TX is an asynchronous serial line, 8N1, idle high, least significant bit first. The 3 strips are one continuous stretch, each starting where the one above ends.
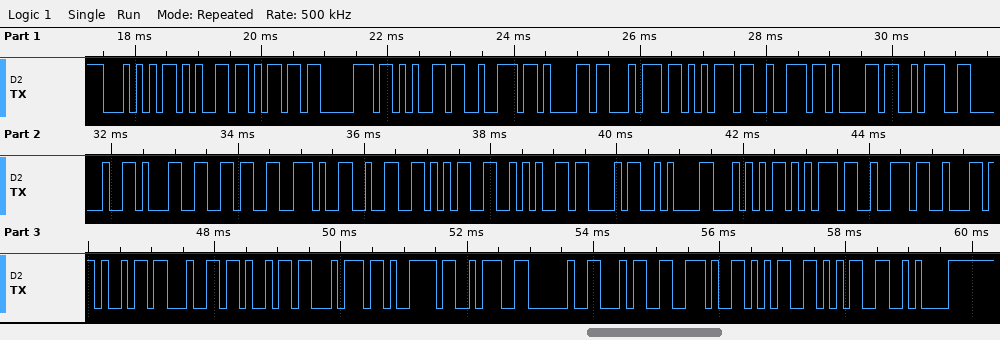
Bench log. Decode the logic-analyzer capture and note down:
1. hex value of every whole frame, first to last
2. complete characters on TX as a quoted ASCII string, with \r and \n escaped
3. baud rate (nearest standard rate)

54 65 6D 70 65 72 61 74 75 72 61 3A 20 31 36 2E 32 35 2A 43 0A 54 75 72 62 69 64 69 74 79 3A 20 34 2E 35 35 0A
"Temperatura: 16.25*C\nTurbidity: 4.55\n"
9600 baud
